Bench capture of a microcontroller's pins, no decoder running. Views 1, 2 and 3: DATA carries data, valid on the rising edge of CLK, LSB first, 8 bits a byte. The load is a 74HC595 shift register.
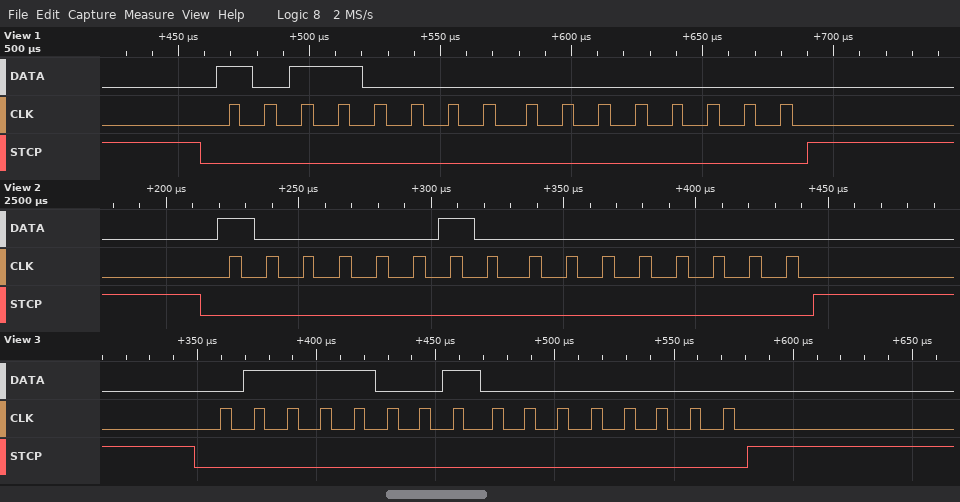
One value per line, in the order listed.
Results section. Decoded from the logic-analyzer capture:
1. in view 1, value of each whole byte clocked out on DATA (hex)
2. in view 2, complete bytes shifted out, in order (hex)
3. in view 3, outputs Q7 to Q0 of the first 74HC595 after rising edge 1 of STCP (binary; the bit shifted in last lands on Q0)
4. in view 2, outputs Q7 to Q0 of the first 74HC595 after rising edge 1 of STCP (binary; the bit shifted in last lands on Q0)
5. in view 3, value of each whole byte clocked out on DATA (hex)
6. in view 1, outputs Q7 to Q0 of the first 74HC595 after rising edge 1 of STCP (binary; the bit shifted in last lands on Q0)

0x0D 0x00
41 00
00000000
00000000
9E 00
00000000
